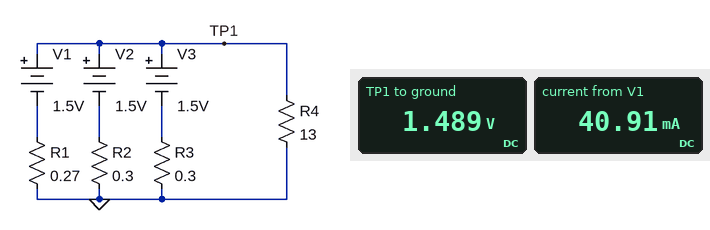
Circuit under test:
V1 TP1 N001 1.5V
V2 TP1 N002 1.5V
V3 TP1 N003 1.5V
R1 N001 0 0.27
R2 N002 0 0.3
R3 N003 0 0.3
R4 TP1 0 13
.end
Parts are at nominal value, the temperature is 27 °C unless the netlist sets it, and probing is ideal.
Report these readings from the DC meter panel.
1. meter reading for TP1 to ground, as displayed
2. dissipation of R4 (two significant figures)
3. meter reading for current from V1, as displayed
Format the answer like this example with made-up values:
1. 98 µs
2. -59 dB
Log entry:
1. 1.489 V
2. 170 mW
3. 40.91 mA
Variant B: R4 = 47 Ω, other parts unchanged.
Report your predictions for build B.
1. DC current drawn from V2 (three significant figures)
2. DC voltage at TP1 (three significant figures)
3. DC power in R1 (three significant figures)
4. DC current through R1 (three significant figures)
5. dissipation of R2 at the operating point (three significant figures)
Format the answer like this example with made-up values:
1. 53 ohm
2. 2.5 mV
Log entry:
1. 10.2 mA
2. 1.50 V
3. 34.9 µW
4. 11.4 mA
5. 31.4 µW
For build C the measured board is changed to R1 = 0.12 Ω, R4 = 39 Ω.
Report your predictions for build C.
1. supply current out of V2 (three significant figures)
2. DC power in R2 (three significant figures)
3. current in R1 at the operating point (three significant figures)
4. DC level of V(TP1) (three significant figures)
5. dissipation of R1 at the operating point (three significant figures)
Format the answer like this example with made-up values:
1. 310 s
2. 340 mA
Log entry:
1. 8.53 mA
2. 21.8 µW
3. 21.3 mA
4. 1.50 V
5. 54.6 µW
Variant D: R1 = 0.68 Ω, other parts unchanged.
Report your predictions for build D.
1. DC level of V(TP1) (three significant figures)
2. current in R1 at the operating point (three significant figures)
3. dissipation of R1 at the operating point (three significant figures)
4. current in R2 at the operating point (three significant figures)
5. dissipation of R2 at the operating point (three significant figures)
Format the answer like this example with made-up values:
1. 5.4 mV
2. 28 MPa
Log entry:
1. 1.49 V
2. 20.7 mA
3. 290 µW
4. 46.8 mA
5. 658 µW
